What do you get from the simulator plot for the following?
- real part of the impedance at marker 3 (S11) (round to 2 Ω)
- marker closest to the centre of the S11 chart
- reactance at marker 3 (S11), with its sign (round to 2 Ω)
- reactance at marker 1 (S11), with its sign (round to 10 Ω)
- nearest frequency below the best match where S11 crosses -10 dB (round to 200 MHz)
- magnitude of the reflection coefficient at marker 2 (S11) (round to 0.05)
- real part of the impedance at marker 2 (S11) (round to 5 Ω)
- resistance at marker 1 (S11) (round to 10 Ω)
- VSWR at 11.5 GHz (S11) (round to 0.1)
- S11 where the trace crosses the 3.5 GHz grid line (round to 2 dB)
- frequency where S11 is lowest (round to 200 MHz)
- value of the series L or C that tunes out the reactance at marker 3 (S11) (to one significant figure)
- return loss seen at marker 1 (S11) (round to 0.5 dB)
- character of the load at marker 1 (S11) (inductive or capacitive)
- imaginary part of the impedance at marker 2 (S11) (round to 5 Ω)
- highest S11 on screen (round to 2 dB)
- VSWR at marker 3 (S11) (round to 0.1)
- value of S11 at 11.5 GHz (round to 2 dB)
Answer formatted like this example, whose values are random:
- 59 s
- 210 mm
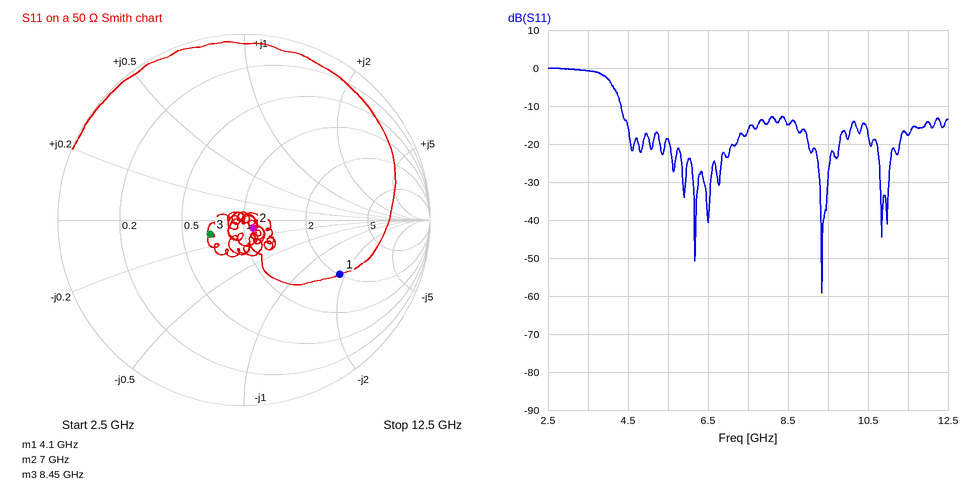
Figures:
- 34 Ω
- marker 2
- -6 Ω
- -90 Ω
- 4.4 GHz
- 0.05
- 55 Ω
- 100 Ω
- 1.3
- 0 dB
- 9.4 GHz
- 100 pH
- 4.5 dB
- capacitive
- -5 Ω
- 0 dB
- 1.5
- -18 dB
